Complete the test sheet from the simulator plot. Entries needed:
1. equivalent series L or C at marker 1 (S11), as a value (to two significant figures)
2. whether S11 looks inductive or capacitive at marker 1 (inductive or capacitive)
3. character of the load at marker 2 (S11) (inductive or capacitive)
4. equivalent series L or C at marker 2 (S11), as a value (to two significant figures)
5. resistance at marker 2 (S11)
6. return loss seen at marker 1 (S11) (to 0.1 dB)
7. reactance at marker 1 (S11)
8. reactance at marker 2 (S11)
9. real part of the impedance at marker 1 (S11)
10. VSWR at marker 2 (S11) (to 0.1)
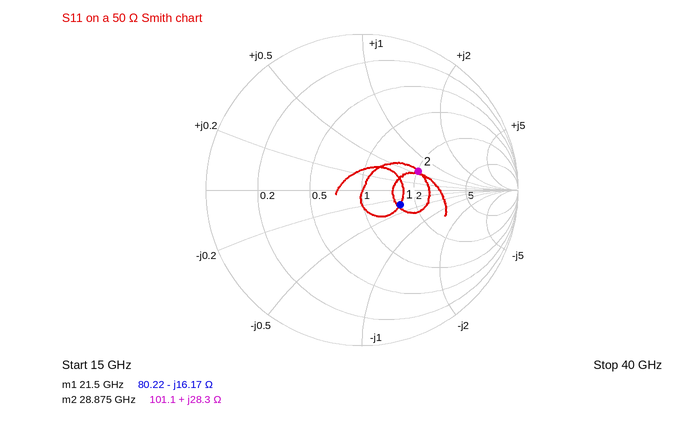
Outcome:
460 fF
capacitive
inductive
160 pH
101.1 Ω
11.7 dB
-16.17 Ω
+28.3 Ω
80.22 Ω
2.2
